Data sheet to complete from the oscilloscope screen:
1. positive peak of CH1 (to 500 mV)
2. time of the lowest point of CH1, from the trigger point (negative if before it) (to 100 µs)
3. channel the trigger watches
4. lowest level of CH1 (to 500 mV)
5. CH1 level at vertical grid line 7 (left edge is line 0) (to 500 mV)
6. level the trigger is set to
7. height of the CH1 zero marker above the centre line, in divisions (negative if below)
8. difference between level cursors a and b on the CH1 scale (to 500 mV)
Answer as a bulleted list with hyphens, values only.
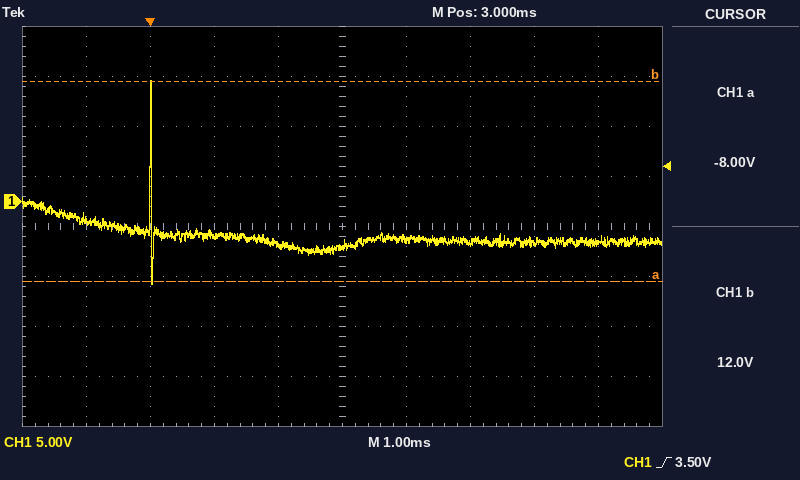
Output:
- 12.0 V
- 0.0 ms
- CH1
- -8.0 V
- -4.0 V
- 3.50 V
- +0.5 div
- 20.0 V
